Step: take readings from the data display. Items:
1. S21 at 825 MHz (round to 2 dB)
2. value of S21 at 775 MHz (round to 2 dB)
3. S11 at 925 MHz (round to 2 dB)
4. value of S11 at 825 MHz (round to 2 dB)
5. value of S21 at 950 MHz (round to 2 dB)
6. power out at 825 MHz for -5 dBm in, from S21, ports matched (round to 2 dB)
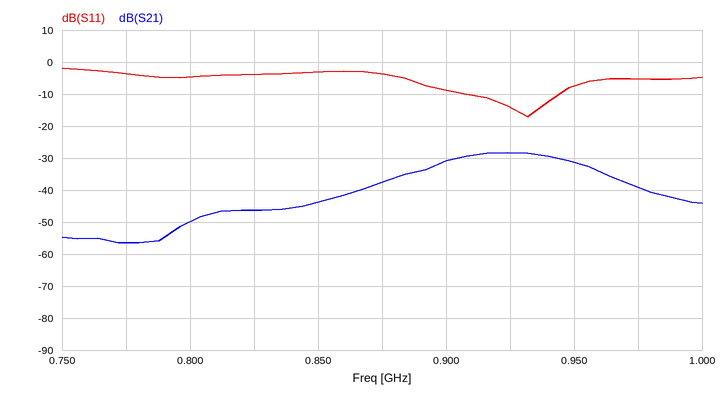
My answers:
-46 dB
-56 dB
-14 dB
-4 dB
-32 dB
-52 dBm
